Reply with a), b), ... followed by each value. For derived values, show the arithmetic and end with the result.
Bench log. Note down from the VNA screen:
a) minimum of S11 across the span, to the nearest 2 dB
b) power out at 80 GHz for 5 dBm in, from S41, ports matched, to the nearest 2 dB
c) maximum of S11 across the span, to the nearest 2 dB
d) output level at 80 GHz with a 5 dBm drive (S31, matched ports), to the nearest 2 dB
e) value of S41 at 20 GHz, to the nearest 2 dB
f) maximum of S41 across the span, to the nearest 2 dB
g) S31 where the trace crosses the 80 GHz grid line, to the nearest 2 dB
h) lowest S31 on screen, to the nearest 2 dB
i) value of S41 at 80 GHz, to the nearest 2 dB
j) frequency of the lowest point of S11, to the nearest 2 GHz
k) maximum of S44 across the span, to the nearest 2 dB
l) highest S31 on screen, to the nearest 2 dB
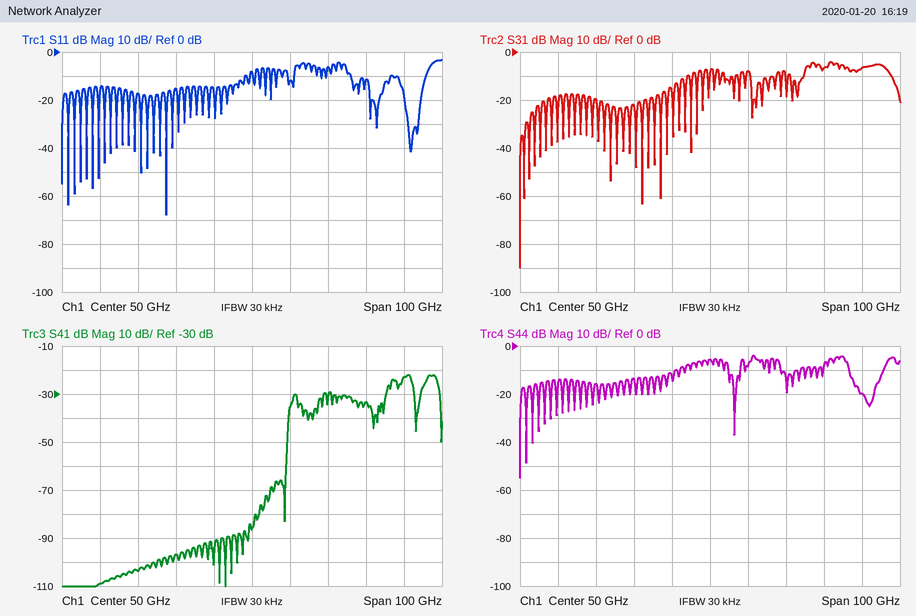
a) -68 dB
b) 5 dBm + (-34 dB) = -28 dBm
c) -4 dB
d) 5 dBm + (-6 dB) = -2 dBm
e) -104 dB
f) -22 dB
g) -6 dB
h) -90 dB
i) -34 dB
j) 28 GHz
k) -4 dB
l) -4 dB
